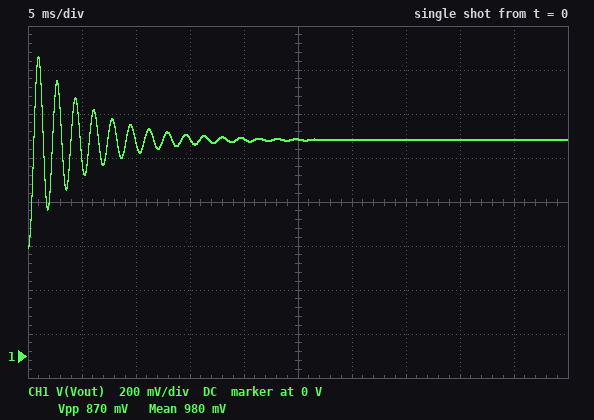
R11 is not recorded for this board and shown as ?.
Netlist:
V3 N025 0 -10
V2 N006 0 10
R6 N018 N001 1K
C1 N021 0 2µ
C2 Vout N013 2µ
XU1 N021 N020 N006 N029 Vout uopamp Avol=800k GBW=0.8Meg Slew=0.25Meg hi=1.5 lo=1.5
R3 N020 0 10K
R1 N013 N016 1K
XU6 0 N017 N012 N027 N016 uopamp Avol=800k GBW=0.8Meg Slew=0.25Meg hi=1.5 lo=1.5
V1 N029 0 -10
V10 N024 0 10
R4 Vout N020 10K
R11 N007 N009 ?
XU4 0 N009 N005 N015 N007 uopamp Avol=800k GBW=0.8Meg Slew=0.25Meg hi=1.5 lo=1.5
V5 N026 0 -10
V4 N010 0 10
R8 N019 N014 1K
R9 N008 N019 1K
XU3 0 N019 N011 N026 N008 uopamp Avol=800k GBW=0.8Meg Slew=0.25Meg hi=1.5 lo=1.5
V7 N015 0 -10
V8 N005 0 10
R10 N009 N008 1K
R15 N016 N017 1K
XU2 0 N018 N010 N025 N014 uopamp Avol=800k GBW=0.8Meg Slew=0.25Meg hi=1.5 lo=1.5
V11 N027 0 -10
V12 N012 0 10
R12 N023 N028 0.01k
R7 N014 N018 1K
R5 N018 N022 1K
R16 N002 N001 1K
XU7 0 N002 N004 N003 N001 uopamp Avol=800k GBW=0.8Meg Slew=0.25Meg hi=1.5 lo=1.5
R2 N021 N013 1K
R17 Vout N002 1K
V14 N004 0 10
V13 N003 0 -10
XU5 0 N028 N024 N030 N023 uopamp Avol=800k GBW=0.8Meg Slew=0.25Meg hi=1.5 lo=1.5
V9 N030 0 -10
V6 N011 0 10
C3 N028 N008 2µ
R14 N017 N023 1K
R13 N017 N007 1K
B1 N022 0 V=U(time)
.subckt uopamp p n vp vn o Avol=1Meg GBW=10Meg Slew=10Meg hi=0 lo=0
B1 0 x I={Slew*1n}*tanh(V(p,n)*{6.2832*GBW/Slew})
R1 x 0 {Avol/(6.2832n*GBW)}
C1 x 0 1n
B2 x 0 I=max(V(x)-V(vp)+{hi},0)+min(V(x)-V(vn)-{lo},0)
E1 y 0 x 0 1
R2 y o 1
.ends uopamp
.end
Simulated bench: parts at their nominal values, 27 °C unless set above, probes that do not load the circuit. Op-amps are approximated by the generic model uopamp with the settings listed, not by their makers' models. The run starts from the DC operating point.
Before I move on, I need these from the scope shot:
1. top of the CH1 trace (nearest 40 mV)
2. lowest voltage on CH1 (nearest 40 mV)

1.36 V
480 mV
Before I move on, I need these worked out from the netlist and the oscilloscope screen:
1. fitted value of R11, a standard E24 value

27 kΩ
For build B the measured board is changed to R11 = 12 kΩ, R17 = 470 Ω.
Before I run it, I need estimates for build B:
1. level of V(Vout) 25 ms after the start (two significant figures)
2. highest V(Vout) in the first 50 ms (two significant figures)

460 mV
650 mV
